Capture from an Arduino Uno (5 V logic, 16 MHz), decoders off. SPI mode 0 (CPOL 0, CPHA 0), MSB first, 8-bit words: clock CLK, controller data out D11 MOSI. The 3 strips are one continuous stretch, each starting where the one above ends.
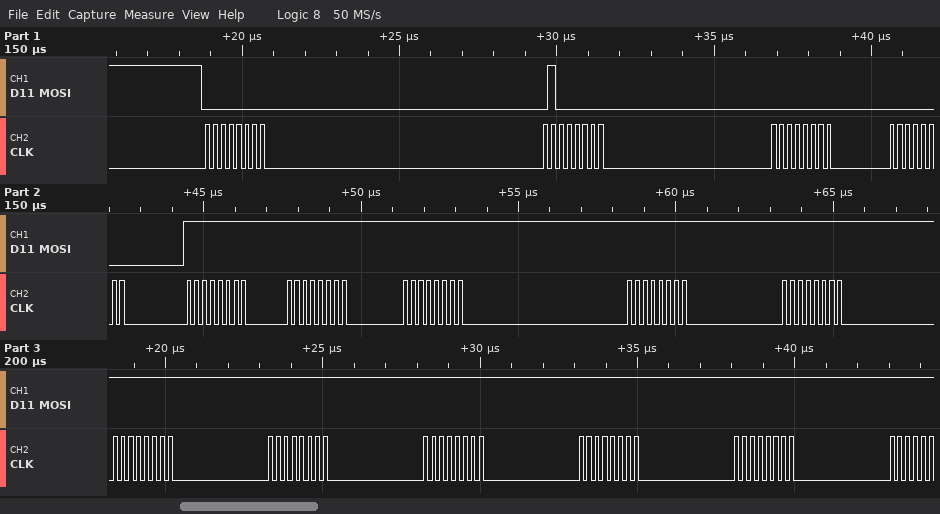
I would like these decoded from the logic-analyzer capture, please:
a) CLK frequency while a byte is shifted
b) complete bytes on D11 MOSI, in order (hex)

4 MHz
0x00 0x40 0x00 0x00 0xFF 0xFF 0xFF 0xFF 0xFF 0xFF 0xFF 0xFF 0xFF 0xFF
